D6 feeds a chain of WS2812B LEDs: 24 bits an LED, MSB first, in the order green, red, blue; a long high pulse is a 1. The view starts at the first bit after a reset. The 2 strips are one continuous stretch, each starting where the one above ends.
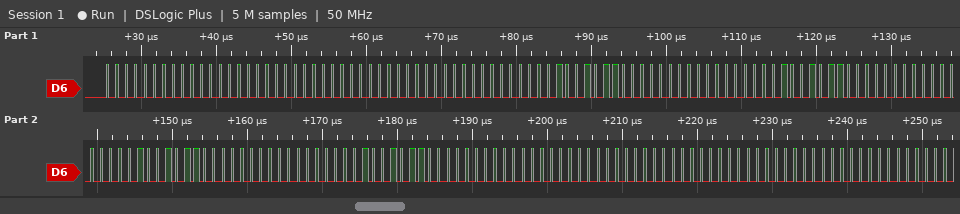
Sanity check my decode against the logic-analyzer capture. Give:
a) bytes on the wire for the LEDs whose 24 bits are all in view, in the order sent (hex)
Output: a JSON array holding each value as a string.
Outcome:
["00 00 00 00 00 00 96 00 00 96 00 00 96 00 00 96 00 00 00 00 00"]
